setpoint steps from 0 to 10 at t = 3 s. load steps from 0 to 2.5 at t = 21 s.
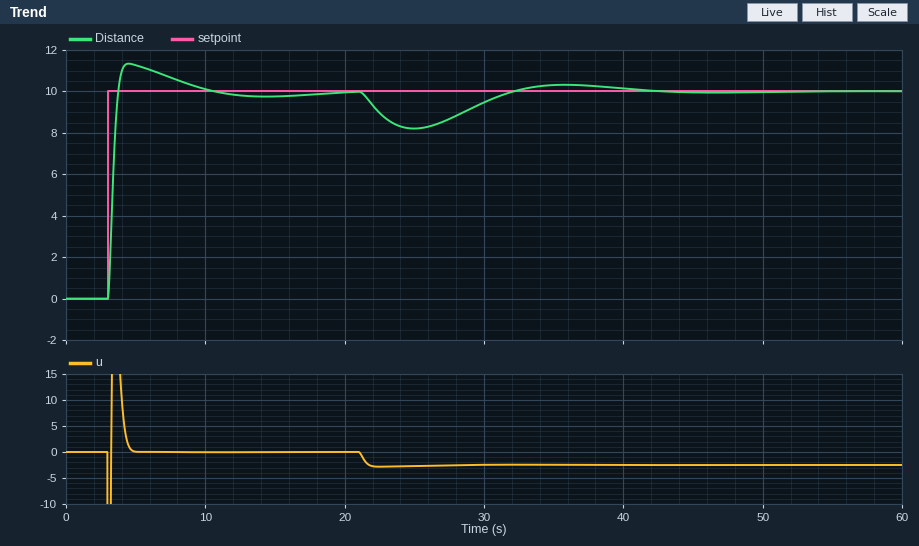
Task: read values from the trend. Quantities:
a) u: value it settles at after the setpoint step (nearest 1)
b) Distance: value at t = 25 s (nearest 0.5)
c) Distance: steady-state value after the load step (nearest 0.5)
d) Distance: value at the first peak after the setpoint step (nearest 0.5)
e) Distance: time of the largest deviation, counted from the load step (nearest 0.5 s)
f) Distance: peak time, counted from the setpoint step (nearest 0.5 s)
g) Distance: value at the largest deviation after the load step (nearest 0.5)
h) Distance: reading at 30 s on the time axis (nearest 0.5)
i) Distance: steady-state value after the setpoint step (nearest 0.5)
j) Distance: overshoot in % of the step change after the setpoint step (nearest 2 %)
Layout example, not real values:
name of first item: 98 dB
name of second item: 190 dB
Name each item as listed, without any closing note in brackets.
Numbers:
u: value it settles at after the setpoint step: 0
Distance: value at t = 25 s: 8.0
Distance: steady-state value after the load step: 10.0
Distance: value at the first peak after the setpoint step: 11.5
Distance: time of the largest deviation, counted from the load step: 4.0 s
Distance: peak time, counted from the setpoint step: 1.5 s
Distance: value at the largest deviation after the load step: 8.0
Distance: reading at 30 s on the time axis: 9.5
Distance: steady-state value after the setpoint step: 10.0
Distance: overshoot in % of the step change after the setpoint step: 14 %
